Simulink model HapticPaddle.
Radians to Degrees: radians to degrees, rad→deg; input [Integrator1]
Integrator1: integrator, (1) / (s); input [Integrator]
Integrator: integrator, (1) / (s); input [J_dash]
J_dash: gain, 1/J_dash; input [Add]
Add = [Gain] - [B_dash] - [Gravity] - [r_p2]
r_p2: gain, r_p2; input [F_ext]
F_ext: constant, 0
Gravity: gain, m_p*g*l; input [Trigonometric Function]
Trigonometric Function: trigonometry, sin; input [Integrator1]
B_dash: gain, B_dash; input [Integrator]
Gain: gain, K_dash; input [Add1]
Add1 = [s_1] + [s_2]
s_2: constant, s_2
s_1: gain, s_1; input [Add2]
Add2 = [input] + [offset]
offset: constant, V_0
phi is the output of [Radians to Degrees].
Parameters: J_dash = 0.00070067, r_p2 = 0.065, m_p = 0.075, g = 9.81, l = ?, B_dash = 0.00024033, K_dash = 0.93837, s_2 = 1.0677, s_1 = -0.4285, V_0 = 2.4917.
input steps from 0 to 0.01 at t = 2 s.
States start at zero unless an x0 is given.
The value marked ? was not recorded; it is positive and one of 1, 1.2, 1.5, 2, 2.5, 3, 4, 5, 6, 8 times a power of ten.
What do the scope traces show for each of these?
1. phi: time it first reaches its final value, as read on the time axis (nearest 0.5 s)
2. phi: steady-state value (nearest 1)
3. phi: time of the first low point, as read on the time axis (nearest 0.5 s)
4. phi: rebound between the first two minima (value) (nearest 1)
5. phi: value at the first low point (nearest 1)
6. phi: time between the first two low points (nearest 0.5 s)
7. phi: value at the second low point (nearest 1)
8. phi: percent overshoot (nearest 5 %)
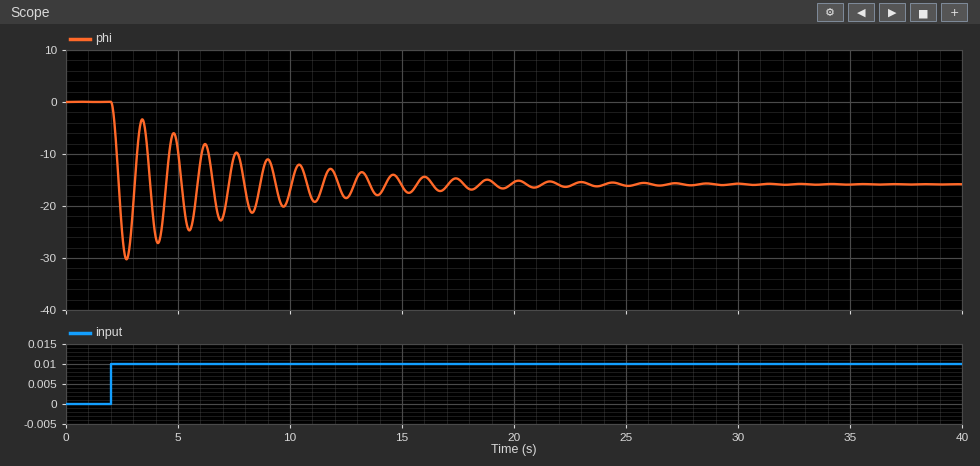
2.5 s
-16
2.5 s
-3
-30
1.5 s
-27
90 %
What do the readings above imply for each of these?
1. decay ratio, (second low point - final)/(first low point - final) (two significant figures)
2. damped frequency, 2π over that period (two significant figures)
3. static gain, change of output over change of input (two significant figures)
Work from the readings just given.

0.79
4.2 rad/s
-1600
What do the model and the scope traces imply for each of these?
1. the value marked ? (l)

0.02
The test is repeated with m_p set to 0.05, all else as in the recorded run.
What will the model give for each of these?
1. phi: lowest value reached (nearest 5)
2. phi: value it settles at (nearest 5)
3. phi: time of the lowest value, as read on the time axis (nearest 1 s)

-45
-25
3 s
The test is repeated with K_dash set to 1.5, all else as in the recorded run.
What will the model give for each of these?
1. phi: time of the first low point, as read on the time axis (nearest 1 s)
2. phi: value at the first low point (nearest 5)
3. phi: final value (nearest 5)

3 s
-50
-25
